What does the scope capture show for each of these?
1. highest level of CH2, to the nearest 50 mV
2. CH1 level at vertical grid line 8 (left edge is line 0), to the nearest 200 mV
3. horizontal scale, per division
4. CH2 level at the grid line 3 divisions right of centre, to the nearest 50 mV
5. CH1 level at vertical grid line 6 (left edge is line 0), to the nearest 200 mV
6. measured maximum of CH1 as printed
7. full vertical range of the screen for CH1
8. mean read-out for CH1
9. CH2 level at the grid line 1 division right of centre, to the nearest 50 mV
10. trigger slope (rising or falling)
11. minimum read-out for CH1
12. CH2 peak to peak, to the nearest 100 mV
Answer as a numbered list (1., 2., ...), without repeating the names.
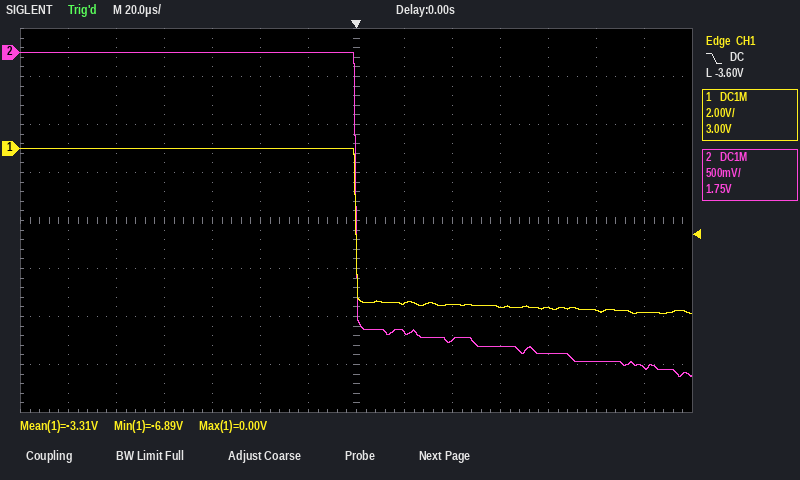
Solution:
1. 0 mV
2. -6.4 V
3. 20 µs
4. -3.05 V
5. 0.0 V
6. 0.00 V
7. 16 V
8. -3.31 V
9. -2.90 V
10. falling
11. -6.89 V
12. 3.40 V
